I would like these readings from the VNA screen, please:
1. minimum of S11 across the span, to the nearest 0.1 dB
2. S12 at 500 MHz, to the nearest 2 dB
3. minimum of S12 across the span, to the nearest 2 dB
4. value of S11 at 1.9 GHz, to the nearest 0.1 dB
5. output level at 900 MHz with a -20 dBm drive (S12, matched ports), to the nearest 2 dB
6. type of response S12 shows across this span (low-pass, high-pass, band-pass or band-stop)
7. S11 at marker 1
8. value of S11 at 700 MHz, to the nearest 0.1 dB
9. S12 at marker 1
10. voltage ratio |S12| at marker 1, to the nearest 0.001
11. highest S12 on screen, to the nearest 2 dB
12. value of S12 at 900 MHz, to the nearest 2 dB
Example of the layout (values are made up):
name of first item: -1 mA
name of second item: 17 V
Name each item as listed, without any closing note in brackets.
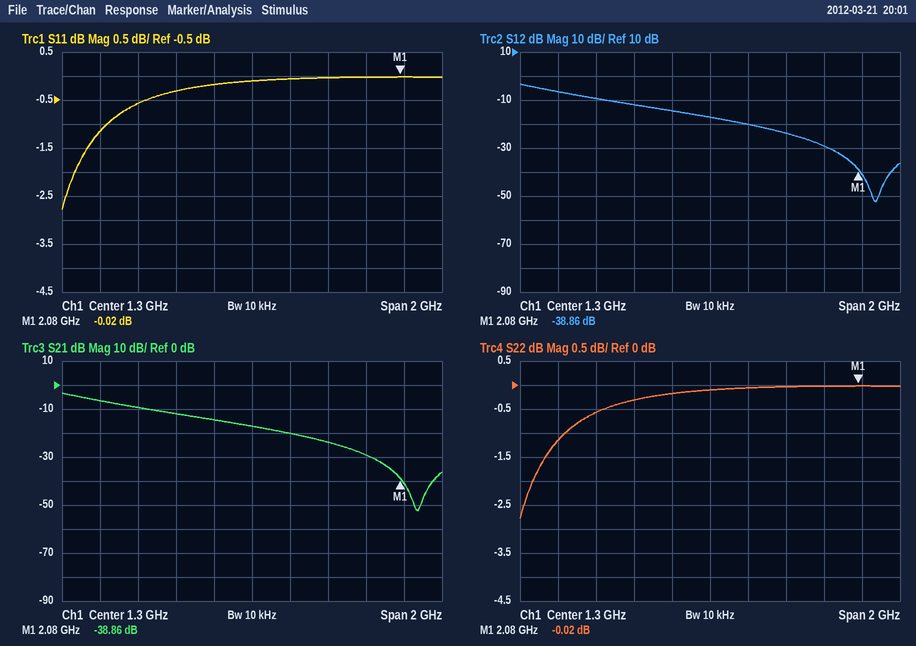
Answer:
minimum of S11 across the span, to the nearest 0.1 dB: -2.8 dB
S12 at 500 MHz, to the nearest 2 dB: -6 dB
minimum of S12 across the span, to the nearest 2 dB: -52 dB
value of S11 at 1.9 GHz, to the nearest 0.1 dB: 0.0 dB
output level at 900 MHz with a -20 dBm drive (S12, matched ports), to the nearest 2 dB: -32 dBm
type of response S12 shows across this span: low-pass
S11 at marker 1: -0.02 dB
value of S11 at 700 MHz, to the nearest 0.1 dB: -0.6 dB
S12 at marker 1: -38.86 dB
voltage ratio |S12| at marker 1, to the nearest 0.001: 0.011
highest S12 on screen, to the nearest 2 dB: -4 dB
value of S12 at 900 MHz, to the nearest 2 dB: -12 dB
